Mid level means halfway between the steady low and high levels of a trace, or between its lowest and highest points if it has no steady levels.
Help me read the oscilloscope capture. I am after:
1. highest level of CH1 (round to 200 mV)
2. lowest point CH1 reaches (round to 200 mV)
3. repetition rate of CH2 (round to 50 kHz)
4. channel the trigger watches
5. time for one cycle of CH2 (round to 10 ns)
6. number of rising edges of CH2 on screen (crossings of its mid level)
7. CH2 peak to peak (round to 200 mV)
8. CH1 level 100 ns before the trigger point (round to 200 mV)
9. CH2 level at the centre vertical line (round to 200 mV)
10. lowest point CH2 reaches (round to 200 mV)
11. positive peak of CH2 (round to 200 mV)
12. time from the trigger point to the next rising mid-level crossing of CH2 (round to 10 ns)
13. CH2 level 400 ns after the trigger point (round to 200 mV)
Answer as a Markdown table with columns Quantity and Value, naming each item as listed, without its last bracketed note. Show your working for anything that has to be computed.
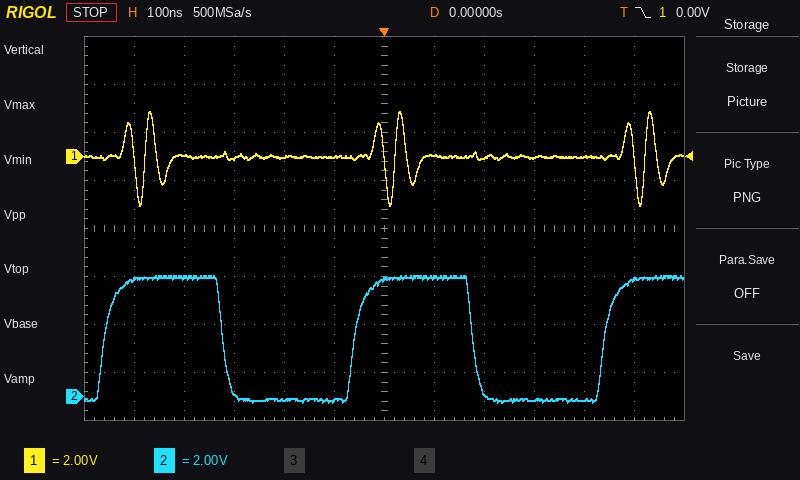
| Quantity | Value |
|---|---|
| highest level of CH1 | 1.8 V |
| lowest point CH1 reaches | -2.0 V |
| repetition rate of CH2 | 1 / 500 ns ≈ 2.00 MHz |
| channel the trigger watches | CH1 |
| time for one cycle of CH2 | 500 ns |
| number of rising edges of CH2 on screen | 3 |
| CH2 peak to peak | 5.0 V − (-200 mV) = 5.2 V |
| CH1 level 100 ns before the trigger point | 0.0 V |
| CH2 level at the centre vertical line | 4.8 V |
| lowest point CH2 reaches | -200 mV |
| positive peak of CH2 | 5.0 V |
| time from the trigger point to the next rising mid-level crossing of CH2 | 440 ns |
| CH2 level 400 ns after the trigger point | -200 mV |
